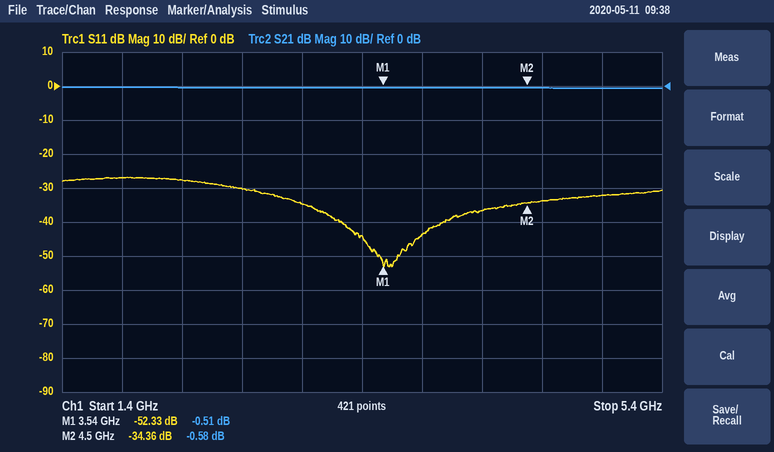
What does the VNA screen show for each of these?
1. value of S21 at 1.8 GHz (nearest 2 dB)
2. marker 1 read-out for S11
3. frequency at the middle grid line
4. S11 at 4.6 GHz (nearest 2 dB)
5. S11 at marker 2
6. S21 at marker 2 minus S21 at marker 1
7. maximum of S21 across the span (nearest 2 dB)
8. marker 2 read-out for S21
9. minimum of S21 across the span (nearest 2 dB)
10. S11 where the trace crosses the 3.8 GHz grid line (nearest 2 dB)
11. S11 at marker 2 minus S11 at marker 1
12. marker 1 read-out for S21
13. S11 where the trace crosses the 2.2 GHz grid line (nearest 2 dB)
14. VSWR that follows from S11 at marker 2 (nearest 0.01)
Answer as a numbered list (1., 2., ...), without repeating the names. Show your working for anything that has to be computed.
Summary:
1. 0 dB
2. -52.33 dB
3. 3.4 GHz
4. -34 dB
5. -34.36 dB
6. -0.58 − (-0.51) = -0.07 dB
7. 0 dB
8. -0.58 dB
9. 0 dB
10. -44 dB
11. -34.36 − (-52.33) = 17.97 dB
12. -0.51 dB
13. -28 dB
14. (1 + 0.0191)/(1 − 0.0191) ≈ 1.04
